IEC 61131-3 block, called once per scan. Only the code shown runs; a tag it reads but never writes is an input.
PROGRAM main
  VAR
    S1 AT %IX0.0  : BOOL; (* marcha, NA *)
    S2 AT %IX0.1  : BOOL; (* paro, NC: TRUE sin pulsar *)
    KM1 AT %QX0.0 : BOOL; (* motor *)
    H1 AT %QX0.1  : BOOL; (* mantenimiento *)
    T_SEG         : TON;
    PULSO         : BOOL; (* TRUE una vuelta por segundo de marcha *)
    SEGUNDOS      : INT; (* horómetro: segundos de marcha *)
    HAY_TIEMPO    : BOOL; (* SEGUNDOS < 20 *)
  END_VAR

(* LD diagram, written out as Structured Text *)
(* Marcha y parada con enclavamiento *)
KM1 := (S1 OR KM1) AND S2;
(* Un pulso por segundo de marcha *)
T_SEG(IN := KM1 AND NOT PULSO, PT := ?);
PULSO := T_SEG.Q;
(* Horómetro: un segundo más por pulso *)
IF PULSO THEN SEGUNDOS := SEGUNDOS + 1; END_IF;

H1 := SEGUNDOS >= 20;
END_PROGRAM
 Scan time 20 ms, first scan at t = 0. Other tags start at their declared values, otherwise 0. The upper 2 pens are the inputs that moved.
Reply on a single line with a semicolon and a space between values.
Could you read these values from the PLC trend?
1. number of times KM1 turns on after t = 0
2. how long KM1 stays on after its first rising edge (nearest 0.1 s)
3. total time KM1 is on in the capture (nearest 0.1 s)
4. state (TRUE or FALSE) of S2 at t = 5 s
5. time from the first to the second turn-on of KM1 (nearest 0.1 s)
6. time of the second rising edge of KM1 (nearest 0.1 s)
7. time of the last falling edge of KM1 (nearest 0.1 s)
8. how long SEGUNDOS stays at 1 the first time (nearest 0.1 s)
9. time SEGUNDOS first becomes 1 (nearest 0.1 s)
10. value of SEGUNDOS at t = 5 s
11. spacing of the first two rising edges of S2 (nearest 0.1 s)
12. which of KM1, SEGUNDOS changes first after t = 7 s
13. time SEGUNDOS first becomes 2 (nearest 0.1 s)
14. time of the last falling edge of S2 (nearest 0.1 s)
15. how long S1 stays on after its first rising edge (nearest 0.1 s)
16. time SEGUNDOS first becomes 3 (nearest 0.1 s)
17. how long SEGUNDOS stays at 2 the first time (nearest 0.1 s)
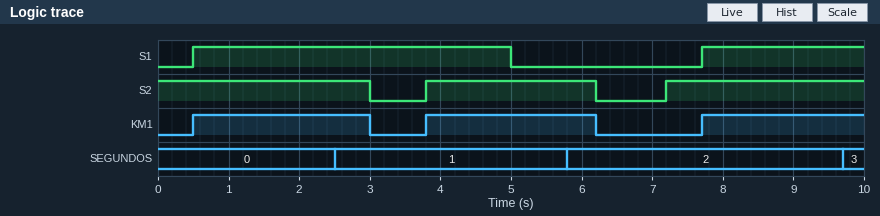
3; 2.5 s; 7.2 s; TRUE; 3.3 s; 3.8 s; 6.2 s; 3.3 s; 2.5 s; 1; 3.4 s; KM1; 5.8 s; 6.2 s; 4.5 s; 9.7 s; 3.9 s
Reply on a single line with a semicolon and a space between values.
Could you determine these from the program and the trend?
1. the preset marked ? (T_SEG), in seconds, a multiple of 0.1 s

2.0 s
